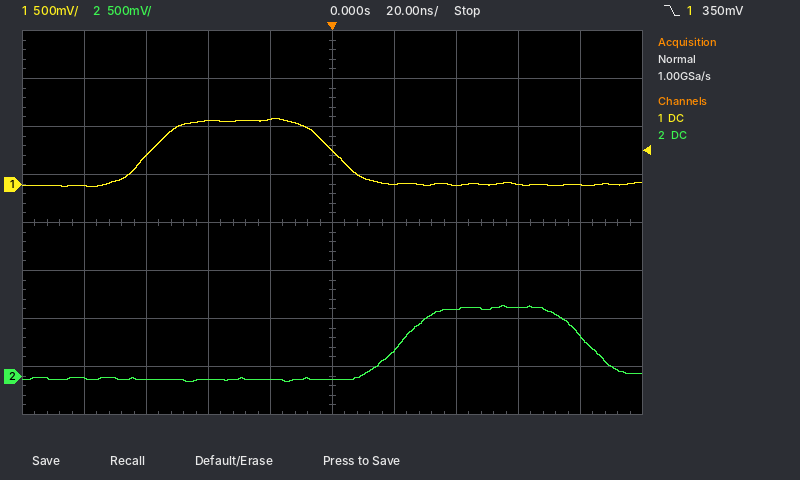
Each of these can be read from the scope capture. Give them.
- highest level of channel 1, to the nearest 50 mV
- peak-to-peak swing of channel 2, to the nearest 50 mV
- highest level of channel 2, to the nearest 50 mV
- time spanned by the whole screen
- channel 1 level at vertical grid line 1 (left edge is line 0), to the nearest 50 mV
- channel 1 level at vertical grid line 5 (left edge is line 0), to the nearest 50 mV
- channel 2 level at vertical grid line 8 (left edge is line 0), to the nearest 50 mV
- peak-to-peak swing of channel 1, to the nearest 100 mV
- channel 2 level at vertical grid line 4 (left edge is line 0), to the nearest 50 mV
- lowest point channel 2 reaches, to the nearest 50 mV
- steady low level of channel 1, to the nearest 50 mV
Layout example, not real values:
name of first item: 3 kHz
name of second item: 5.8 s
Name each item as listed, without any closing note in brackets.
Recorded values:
highest level of channel 1, to the nearest 50 mV: 700 mV
peak-to-peak swing of channel 2, to the nearest 50 mV: 800 mV
highest level of channel 2, to the nearest 50 mV: 750 mV
time spanned by the whole screen: 200 ns
channel 1 level at vertical grid line 1 (left edge is line 0), to the nearest 50 mV: 0 mV
channel 1 level at vertical grid line 5 (left edge is line 0), to the nearest 50 mV: 350 mV
channel 2 level at vertical grid line 8 (left edge is line 0), to the nearest 50 mV: 700 mV
peak-to-peak swing of channel 1, to the nearest 100 mV: 700 mV
channel 2 level at vertical grid line 4 (left edge is line 0), to the nearest 50 mV: -50 mV
lowest point channel 2 reaches, to the nearest 50 mV: -50 mV
steady low level of channel 1, to the nearest 50 mV: 0 mV
